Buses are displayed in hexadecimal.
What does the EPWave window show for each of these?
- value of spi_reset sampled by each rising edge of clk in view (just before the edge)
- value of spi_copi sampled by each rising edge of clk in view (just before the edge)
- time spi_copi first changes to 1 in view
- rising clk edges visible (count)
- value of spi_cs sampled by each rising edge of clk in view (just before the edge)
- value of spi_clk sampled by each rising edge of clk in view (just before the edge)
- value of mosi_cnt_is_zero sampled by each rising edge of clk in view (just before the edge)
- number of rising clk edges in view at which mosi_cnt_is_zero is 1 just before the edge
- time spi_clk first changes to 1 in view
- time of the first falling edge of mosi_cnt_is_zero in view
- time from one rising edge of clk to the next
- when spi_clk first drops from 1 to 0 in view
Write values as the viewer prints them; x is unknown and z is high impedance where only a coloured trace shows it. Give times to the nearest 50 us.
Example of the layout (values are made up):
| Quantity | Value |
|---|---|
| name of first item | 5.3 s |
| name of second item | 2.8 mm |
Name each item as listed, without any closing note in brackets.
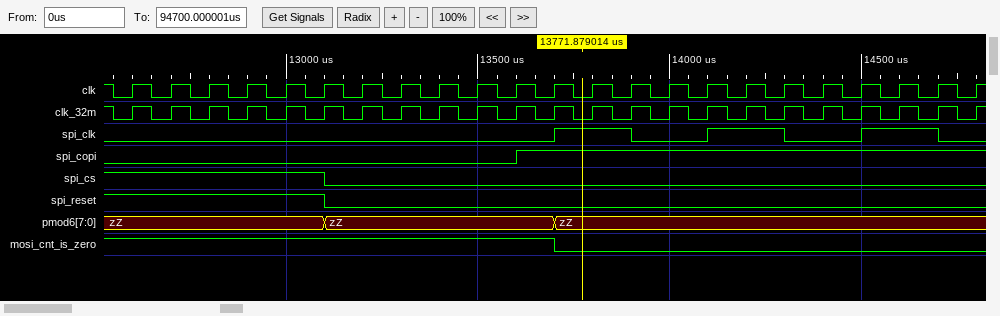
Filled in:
| Quantity | Value |
|---|---|
| value of spi_reset sampled by each rising edge of clk in view | 1 1 1 1 1 1 0 0 0 0 0 0 0 0 0 0 0 0 0 0 0 0 0 |
| value of spi_copi sampled by each rising edge of clk in view | 0 0 0 0 0 0 0 0 0 0 0 1 1 1 1 1 1 1 1 1 1 1 1 |
| time spi_copi first changes to 1 in view | 13600 us |
| rising clk edges visible | 23 |
| value of spi_cs sampled by each rising edge of clk in view | 1 1 1 1 1 1 0 0 0 0 0 0 0 0 0 0 0 0 0 0 0 0 0 |
| value of spi_clk sampled by each rising edge of clk in view | 0 0 0 0 0 0 0 0 0 0 0 0 1 1 0 0 1 1 0 0 1 1 0 |
| value of mosi_cnt_is_zero sampled by each rising edge of clk in view | 1 1 1 1 1 1 1 1 1 1 1 1 0 0 0 0 0 0 0 0 0 0 0 |
| number of rising clk edges in view at which mosi_cnt_is_zero is 1 just before the edge | 12 |
| time spi_clk first changes to 1 in view | 13700 us |
| time of the first falling edge of mosi_cnt_is_zero in view | 13700 us |
| time from one rising edge of clk to the next | 100 us |
| when spi_clk first drops from 1 to 0 in view | 13900 us |
